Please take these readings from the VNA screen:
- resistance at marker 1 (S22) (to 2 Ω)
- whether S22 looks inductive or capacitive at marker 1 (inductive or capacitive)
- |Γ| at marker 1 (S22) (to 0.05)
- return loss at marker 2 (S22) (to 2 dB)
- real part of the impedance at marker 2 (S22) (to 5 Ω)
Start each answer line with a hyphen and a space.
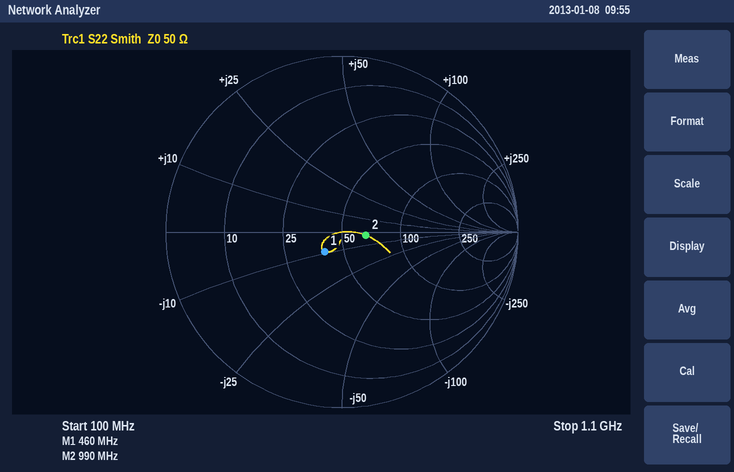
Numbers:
- 40 Ω
- capacitive
- 0.15
- 18 dB
- 65 Ω
